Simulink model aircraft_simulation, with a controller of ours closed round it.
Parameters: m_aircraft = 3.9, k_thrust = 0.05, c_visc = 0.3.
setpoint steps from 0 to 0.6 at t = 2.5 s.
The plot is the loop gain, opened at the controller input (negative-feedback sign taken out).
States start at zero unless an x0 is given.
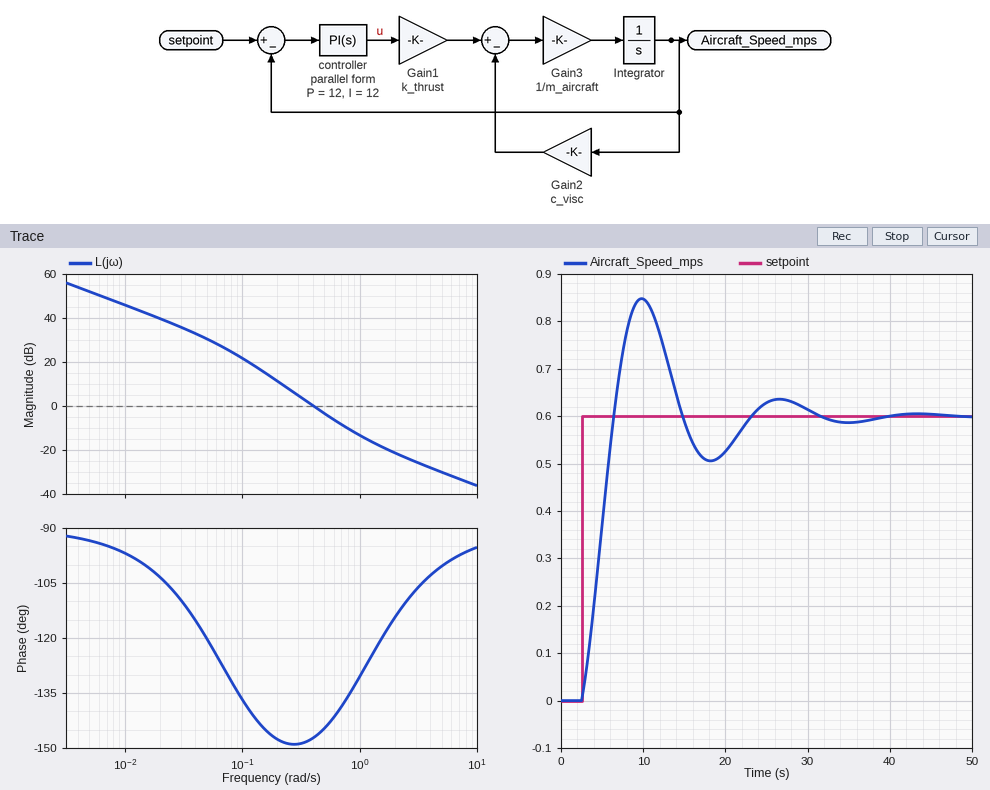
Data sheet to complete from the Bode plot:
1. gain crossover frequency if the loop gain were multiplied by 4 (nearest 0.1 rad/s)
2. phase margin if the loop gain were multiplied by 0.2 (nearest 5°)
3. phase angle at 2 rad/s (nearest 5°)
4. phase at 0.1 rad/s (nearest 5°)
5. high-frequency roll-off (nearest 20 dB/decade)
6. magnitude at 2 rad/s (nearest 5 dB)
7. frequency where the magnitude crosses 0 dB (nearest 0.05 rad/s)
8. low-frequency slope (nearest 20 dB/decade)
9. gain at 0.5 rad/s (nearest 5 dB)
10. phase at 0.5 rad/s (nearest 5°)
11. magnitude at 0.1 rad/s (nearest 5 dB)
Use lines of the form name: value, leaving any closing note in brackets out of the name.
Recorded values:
gain crossover frequency if the loop gain were multiplied by 4: 0.9 rad/s
phase margin if the loop gain were multiplied by 0.2: 35°
phase angle at 2 rad/s: -115°
phase at 0.1 rad/s: -135°
high-frequency roll-off: -20 dB/decade
magnitude at 2 rad/s: -20 dB
frequency where the magnitude crosses 0 dB: 0.40 rad/s
low-frequency slope: -20 dB/decade
gain at 0.5 rad/s: -5 dB
phase at 0.5 rad/s: -145°
magnitude at 0.1 rad/s: 20 dB
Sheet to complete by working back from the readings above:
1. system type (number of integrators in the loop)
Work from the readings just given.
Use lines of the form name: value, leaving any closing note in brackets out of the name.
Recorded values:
system type: 1
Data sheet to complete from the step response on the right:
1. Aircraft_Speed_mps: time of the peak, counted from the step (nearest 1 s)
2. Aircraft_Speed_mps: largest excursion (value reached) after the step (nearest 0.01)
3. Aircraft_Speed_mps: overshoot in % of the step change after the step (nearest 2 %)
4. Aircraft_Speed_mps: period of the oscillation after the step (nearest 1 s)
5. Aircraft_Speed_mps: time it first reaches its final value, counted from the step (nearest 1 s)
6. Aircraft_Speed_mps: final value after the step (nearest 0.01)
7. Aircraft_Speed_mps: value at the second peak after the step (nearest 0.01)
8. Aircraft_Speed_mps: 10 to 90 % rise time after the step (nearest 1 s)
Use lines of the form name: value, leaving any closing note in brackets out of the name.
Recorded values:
Aircraft_Speed_mps: time of the peak, counted from the step: 7 s
Aircraft_Speed_mps: largest excursion (value reached) after the step: 0.85
Aircraft_Speed_mps: overshoot in % of the step change after the step: 42 %
Aircraft_Speed_mps: period of the oscillation after the step: 17 s
Aircraft_Speed_mps: time it first reaches its final value, counted from the step: 4 s
Aircraft_Speed_mps: final value after the step: 0.60
Aircraft_Speed_mps: value at the second peak after the step: 0.64
Aircraft_Speed_mps: 10 to 90 % rise time after the step: 3 s
